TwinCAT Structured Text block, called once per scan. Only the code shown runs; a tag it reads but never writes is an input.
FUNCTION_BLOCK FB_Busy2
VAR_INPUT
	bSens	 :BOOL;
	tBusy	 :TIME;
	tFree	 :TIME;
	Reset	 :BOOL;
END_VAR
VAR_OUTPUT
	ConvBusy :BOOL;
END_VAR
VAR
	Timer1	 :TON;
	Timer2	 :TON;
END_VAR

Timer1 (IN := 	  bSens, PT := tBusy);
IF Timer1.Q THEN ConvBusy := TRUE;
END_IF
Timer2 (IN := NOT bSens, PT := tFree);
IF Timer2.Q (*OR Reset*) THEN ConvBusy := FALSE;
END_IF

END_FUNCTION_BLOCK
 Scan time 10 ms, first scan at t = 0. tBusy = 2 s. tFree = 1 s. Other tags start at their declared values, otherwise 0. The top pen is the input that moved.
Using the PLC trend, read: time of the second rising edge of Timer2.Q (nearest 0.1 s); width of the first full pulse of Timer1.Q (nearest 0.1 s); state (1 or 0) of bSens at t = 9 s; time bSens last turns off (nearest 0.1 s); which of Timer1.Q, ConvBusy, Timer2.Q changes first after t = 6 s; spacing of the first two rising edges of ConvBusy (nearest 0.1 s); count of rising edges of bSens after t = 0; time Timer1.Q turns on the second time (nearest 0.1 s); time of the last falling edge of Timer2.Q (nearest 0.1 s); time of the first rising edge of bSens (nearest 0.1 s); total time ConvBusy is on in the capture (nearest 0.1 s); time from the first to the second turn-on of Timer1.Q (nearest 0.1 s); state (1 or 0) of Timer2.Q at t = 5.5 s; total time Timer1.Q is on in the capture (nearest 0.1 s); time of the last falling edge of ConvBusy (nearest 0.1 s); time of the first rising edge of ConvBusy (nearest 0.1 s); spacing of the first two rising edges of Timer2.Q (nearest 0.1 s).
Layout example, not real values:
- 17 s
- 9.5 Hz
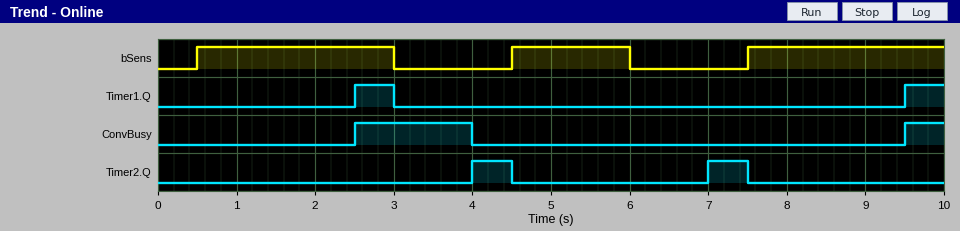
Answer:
- 7.0 s
- 0.5 s
- 1
- 6.0 s
- Timer2.Q
- 7.0 s
- 3
- 9.5 s
- 7.5 s
- 0.5 s
- 2.0 s
- 7.0 s
- 0
- 1.0 s
- 4.0 s
- 2.5 s
- 3.0 s
